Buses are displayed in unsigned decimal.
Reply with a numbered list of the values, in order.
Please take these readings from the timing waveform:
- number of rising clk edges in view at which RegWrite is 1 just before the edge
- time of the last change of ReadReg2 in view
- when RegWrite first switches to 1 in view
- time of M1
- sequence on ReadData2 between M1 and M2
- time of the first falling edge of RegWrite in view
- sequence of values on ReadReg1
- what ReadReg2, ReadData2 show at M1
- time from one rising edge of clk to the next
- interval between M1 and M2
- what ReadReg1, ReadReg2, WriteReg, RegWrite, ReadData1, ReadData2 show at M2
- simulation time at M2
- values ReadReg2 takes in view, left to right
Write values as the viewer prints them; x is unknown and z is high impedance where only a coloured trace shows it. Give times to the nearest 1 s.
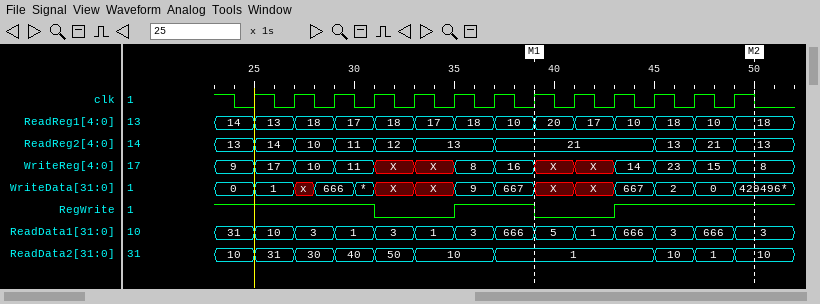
1. 9
2. 49 s
3. 35 s
4. 39 s
5. 1, 10, 1, 10
6. 31 s
7. 14, 13, 18, 17, 18, 17, 18, 10, 20, 17, 10, 18, 10, 18
8. ReadReg2=21, ReadData2=1
9. 2 s
10. 11 s
11. ReadReg1=18, ReadReg2=13, WriteReg=8, RegWrite=1, ReadData1=3, ReadData2=10
12. 50 s
13. 13, 14, 10, 11, 12, 13, 21, 13, 21, 13
